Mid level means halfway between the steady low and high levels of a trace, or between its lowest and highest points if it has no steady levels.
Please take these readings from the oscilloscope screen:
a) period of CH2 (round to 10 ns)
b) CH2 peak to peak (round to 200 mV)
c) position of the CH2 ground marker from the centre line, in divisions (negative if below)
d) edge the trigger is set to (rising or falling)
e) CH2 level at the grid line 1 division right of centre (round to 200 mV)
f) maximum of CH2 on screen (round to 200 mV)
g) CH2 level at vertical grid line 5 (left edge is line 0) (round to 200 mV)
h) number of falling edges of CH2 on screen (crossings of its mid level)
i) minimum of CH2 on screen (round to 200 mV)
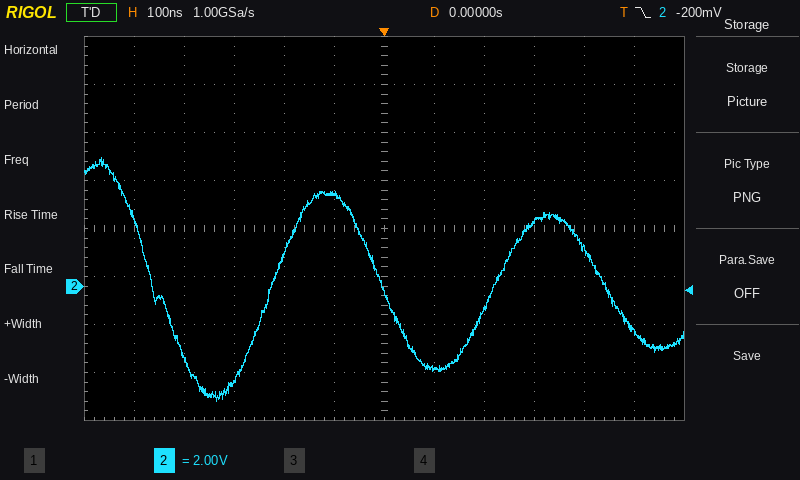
450 ns
10.2 V
-1.2 div
falling
-3.4 V
5.4 V
3.8 V
3
-4.8 V
